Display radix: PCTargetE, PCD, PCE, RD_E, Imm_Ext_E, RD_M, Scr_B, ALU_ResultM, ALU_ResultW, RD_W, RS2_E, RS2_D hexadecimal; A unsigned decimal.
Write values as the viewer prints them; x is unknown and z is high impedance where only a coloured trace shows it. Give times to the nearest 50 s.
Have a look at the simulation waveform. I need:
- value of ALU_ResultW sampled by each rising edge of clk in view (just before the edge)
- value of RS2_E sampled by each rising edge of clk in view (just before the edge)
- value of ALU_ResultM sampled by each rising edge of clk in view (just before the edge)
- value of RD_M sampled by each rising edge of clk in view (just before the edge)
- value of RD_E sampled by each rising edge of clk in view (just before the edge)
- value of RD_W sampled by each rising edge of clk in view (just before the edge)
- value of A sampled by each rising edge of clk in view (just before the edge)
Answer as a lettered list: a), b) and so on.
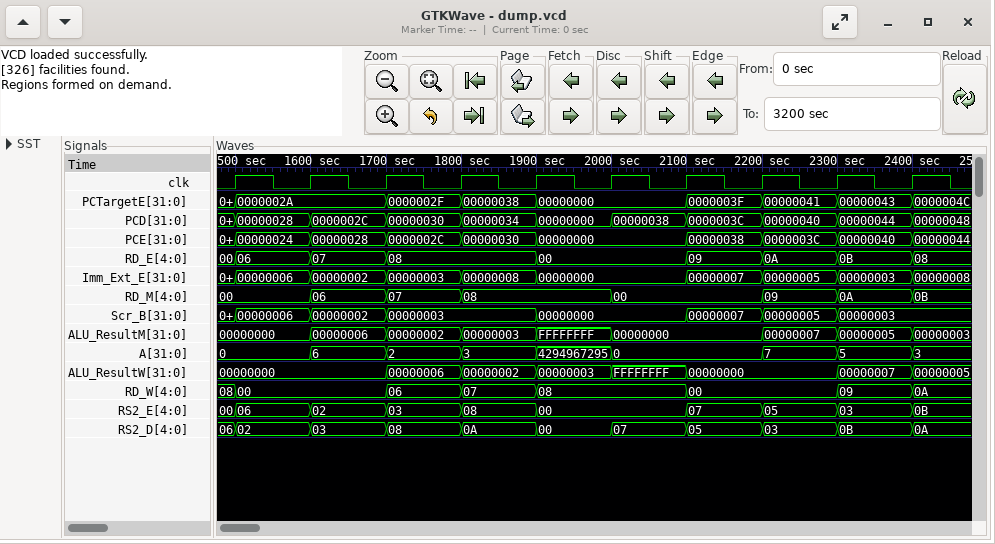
a) 00000000, 00000000, 00000000, 00000006, 00000002, 00000003, FFFFFFFF, 00000000, 00000000, 00000007
b) 00, 06, 02, 03, 08, 00, 00, 07, 05, 03
c) 00000000, 00000000, 00000006, 00000002, 00000003, FFFFFFFF, 00000000, 00000000, 00000007, 00000005
d) 00, 00, 06, 07, 08, 08, 00, 00, 09, 0A
e) 00, 06, 07, 08, 08, 00, 00, 09, 0A, 0B
f) 08, 00, 00, 06, 07, 08, 08, 00, 00, 09
g) 0, 0, 6, 2, 3, 4294967295, 0, 0, 7, 5
